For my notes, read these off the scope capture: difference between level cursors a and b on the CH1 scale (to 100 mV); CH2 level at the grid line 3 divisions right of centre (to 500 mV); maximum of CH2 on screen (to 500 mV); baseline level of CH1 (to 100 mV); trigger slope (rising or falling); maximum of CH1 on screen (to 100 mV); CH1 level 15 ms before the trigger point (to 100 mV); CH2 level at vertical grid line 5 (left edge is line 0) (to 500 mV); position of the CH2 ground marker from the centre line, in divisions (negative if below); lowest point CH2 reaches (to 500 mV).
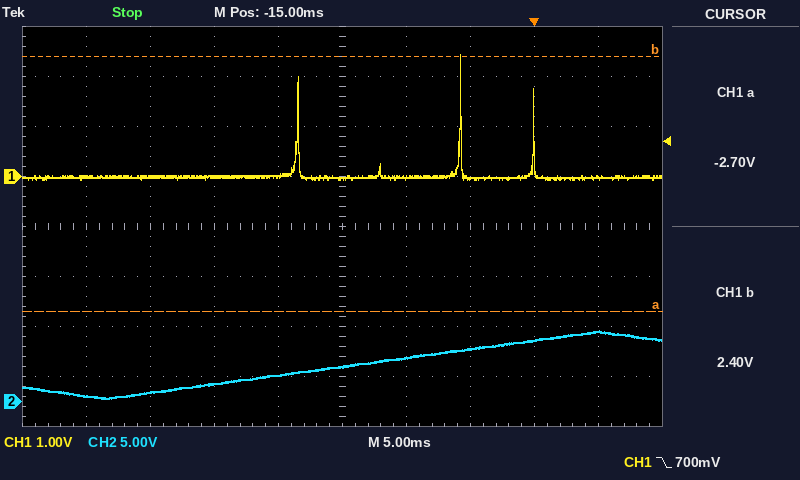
5.1 V
6.0 V
7.0 V
0.0 V
falling
2.4 V
0.0 V
3.5 V
-3.5 div
500 mV
